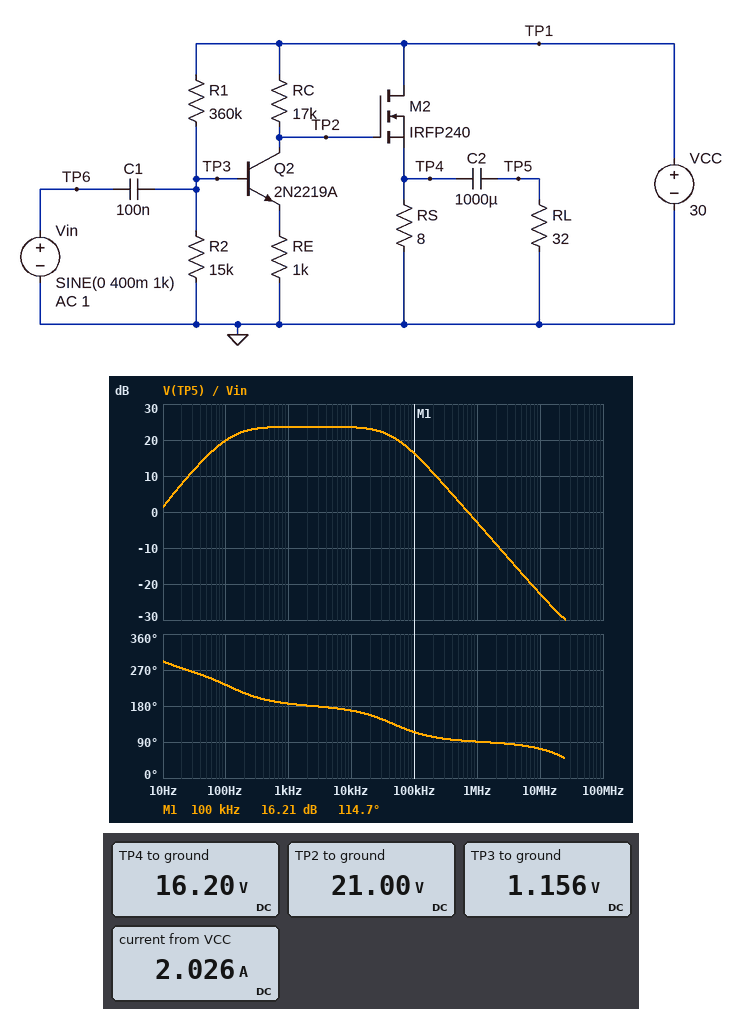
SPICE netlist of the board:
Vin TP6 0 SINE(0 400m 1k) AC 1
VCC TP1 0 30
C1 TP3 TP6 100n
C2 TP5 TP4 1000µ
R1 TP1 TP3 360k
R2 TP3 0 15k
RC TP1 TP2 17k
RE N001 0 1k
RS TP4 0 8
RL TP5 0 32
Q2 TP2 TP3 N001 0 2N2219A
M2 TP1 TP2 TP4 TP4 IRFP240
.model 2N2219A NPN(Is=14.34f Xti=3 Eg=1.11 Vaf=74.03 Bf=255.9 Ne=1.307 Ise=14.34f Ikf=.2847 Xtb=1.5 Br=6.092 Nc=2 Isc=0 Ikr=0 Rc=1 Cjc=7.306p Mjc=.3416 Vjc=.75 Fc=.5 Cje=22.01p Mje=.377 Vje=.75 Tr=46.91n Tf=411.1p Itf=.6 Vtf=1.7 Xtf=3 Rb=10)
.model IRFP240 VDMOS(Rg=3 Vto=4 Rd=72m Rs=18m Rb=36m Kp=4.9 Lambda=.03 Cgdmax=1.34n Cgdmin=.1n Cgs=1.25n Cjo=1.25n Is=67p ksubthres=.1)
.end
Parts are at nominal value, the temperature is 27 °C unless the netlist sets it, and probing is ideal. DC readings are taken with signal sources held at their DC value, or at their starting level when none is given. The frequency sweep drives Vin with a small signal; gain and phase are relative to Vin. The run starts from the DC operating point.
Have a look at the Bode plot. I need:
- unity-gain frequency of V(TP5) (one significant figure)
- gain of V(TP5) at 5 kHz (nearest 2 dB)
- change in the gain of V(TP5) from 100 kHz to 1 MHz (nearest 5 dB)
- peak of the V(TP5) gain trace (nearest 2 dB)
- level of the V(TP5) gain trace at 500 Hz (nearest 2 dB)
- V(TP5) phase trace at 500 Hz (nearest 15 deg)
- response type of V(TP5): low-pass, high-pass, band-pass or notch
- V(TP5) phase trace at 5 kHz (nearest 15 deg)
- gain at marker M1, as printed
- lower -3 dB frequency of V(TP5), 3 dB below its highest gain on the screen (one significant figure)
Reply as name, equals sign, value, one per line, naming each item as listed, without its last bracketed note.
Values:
unity-gain frequency of V(TP5) = 700 kHz
gain of V(TP5) at 5 kHz = 24 dB
change in the gain of V(TP5) from 100 kHz to 1 MHz = -20 dB
peak of the V(TP5) gain trace = 24 dB
level of the V(TP5) gain trace at 500 Hz = 24 dB
V(TP5) phase trace at 500 Hz = 195 deg
response type of V(TP5): low-pass, high-pass, band-pass or notch = band-pass
V(TP5) phase trace at 5 kHz = 180 deg
gain at marker M1, as printed = 16.21 dB
lower -3 dB frequency of V(TP5), 3 dB below its highest gain on the screen = 100 Hz
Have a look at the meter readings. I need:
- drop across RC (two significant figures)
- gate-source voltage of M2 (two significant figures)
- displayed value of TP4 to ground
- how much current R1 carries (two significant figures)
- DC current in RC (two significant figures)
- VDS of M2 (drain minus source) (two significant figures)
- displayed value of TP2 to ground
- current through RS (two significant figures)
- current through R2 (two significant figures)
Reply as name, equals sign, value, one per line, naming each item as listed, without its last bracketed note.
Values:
drop across RC = 9.0 V
gate-source voltage of M2 = 4.8 V
displayed value of TP4 to ground = 16.20 V
how much current R1 carries = 80 µA
DC current in RC = 530 µA
VDS of M2 (drain minus source) = 14 V
displayed value of TP2 to ground = 21.00 V
current through RS = 2.0 A
current through R2 = 77 µA
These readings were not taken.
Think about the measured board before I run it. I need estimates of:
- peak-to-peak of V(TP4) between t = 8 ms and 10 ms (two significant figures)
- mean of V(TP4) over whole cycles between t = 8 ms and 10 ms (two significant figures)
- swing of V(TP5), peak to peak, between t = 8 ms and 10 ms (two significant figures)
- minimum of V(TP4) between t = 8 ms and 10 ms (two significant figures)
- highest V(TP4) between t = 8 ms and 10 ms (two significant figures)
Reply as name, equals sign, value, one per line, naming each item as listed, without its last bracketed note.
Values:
peak-to-peak of V(TP4) between t = 8 ms and 10 ms = 12 V
mean of V(TP4) over whole cycles between t = 8 ms and 10 ms = 16 V
swing of V(TP5), peak to peak, between t = 8 ms and 10 ms = 12 V
minimum of V(TP4) between t = 8 ms and 10 ms = 10 V
highest V(TP4) between t = 8 ms and 10 ms = 22 V
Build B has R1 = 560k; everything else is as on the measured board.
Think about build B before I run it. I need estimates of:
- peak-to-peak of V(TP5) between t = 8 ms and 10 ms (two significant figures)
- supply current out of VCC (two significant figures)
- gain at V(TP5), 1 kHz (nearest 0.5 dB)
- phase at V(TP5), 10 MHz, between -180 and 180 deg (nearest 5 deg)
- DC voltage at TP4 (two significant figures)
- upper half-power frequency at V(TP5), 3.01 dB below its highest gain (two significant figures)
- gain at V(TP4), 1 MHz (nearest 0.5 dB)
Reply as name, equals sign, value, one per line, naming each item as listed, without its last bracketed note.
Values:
peak-to-peak of V(TP5) between t = 8 ms and 10 ms = 8.7 V
supply current out of VCC = 2.8 A
gain at V(TP5), 1 kHz = 23.0 dB
phase at V(TP5), 10 MHz, between -180 and 180 deg = 65 deg
DC voltage at TP4 = 22 V
upper half-power frequency at V(TP5), 3.01 dB below its highest gain = 30 kHz
gain at V(TP4), 1 MHz = -7.5 dB
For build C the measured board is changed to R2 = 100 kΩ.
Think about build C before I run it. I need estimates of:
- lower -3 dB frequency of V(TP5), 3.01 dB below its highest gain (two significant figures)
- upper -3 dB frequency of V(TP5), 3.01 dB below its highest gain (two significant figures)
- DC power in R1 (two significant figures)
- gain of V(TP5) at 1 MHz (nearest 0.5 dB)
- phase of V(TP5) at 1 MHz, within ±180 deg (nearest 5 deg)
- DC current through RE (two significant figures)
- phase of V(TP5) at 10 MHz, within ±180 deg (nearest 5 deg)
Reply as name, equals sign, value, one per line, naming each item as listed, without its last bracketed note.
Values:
lower -3 dB frequency of V(TP5), 3.01 dB below its highest gain = 17 MHz
upper -3 dB frequency of V(TP5), 3.01 dB below its highest gain = 160 MHz
DC power in R1 = 2.1 mW
gain of V(TP5) at 1 MHz = -38.0 dB
phase of V(TP5) at 1 MHz, within ±180 deg = 80 deg
DC current through RE = 1.7 mA
phase of V(TP5) at 10 MHz, within ±180 deg = 60 deg
